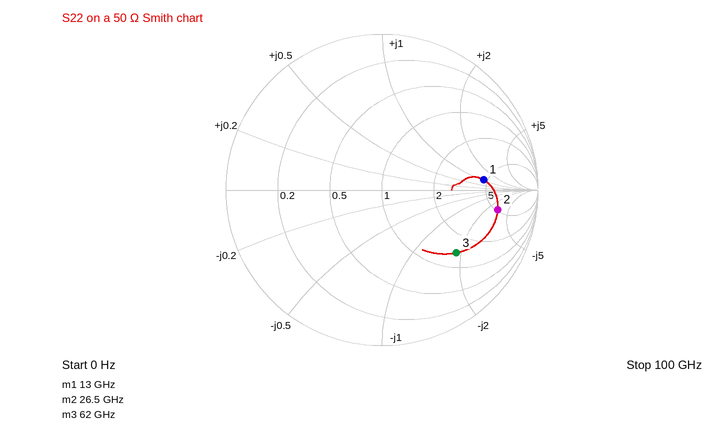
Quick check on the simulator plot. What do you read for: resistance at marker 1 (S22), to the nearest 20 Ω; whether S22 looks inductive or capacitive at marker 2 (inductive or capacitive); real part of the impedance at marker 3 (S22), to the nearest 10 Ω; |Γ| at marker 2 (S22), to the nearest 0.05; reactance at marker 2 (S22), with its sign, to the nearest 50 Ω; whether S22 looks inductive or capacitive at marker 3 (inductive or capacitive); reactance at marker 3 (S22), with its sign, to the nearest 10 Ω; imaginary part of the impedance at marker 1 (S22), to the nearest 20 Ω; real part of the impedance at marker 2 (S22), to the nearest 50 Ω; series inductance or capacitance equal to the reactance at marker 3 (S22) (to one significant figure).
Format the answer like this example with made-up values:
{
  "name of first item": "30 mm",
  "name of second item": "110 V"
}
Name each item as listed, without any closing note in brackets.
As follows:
{
  "resistance at marker 1 (S22), to the nearest 20 Ω": "220 Ω",
  "whether S22 looks inductive or capacitive at marker 2": "capacitive",
  "real part of the impedance at marker 3 (S22), to the nearest 10 Ω": "70 Ω",
  "|Γ| at marker 2 (S22), to the nearest 0.05": "0.75",
  "reactance at marker 2 (S22), with its sign, to the nearest 50 Ω": "-150 Ω",
  "whether S22 looks inductive or capacitive at marker 3": "capacitive",
  "reactance at marker 3 (S22), with its sign, to the nearest 10 Ω": "-90 Ω",
  "imaginary part of the impedance at marker 1 (S22), to the nearest 20 Ω": "+60 Ω",
  "real part of the impedance at marker 2 (S22), to the nearest 50 Ω": "250 Ω",
  "series inductance or capacitance equal to the reactance at marker 3 (S22)": "30 fF"
}
